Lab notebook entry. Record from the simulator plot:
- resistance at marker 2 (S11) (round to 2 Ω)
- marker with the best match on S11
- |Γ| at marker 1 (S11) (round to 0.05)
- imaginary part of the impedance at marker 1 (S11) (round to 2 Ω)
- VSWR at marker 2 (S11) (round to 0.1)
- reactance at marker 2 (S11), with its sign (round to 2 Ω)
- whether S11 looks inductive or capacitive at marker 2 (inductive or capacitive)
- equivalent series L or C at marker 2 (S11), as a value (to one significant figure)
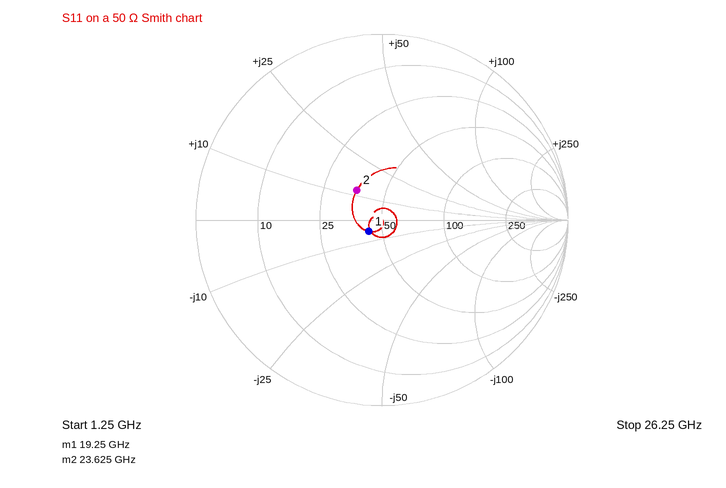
36 Ω
marker 1
0.10
-6 Ω
1.5
+12 Ω
inductive
80 pH
